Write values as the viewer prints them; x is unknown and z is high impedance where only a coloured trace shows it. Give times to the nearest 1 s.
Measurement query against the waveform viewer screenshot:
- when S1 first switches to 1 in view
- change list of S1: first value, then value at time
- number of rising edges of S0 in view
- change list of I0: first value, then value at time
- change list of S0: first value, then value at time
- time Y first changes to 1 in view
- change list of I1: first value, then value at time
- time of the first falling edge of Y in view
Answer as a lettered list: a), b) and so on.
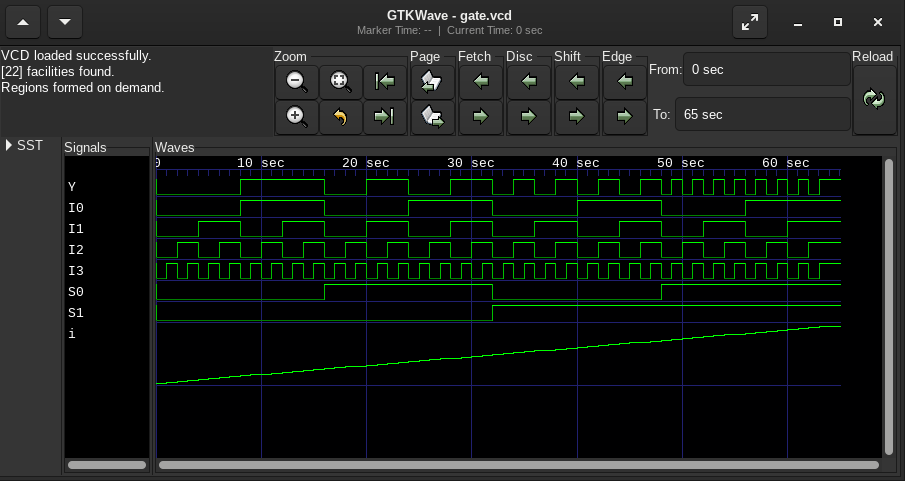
a) 32 s
b) 0, 1 at 32 s
c) 2
d) 0, 1 at 8 s, 0 at 16 s, 1 at 24 s, 0 at 32 s, 1 at 40 s, 0 at 48 s, 1 at 56 s
e) 0, 1 at 16 s, 0 at 32 s, 1 at 48 s
f) 8 s
g) 0, 1 at 4 s, 0 at 8 s, 1 at 12 s, 0 at 16 s, 1 at 20 s, 0 at 24 s, 1 at 28 s, 0 at 32 s, 1 at 36 s, 0 at 40 s, 1 at 44 s, 0 at 48 s, 1 at 52 s, 0 at 56 s, 1 at 60 s
h) 16 s
